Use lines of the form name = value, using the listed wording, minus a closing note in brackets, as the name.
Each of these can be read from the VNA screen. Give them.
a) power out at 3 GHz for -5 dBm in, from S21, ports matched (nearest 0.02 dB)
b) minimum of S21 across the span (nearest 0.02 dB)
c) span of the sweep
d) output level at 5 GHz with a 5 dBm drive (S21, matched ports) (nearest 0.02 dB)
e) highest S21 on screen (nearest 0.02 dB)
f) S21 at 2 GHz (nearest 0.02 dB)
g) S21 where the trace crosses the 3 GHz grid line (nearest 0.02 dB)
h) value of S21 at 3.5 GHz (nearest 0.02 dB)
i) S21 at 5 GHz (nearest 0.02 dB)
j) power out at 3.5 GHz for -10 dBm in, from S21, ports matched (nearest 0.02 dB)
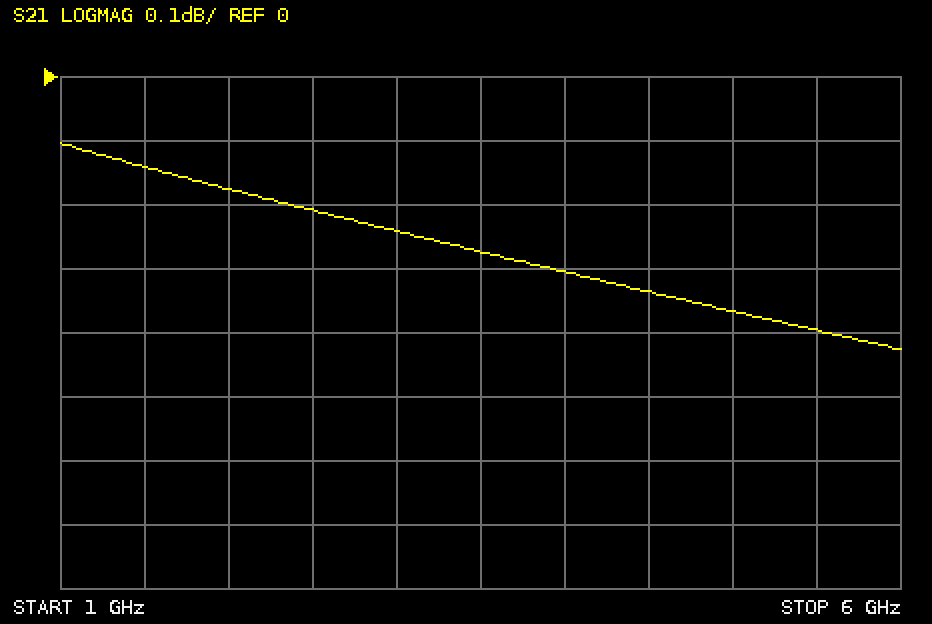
power out at 3 GHz for -5 dBm in, from S21, ports matched = -5.24 dBm
minimum of S21 across the span = -0.42 dB
span of the sweep = 5 GHz
output level at 5 GHz with a 5 dBm drive (S21, matched ports) = 4.64 dBm
highest S21 on screen = -0.10 dB
S21 at 2 GHz = -0.18 dB
S21 where the trace crosses the 3 GHz grid line = -0.24 dB
value of S21 at 3.5 GHz = -0.28 dB
S21 at 5 GHz = -0.36 dB
power out at 3.5 GHz for -10 dBm in, from S21, ports matched = -10.28 dBm
